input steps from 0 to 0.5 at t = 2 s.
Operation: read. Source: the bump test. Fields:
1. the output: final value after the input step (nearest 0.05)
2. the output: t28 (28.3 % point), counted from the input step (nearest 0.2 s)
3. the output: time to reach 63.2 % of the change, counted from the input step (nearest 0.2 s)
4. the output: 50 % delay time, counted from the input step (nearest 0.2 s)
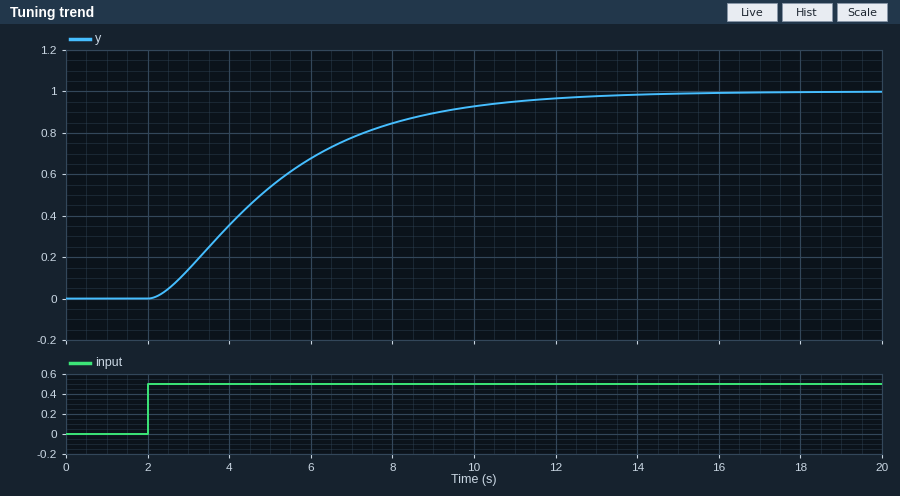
1.00
1.6 s
3.6 s
2.8 s
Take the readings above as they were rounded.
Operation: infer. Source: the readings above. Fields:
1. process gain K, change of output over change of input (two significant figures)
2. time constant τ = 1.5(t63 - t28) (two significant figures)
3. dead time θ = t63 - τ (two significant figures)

2.0
3.0 s
0.60 s
